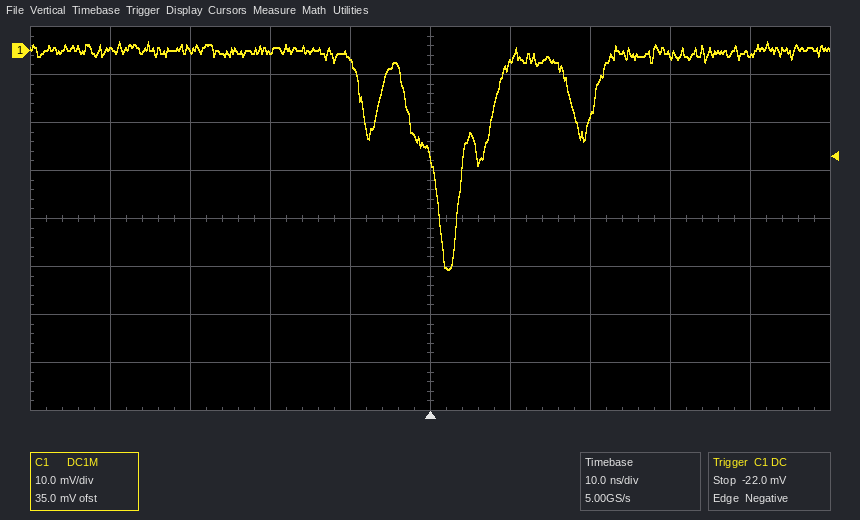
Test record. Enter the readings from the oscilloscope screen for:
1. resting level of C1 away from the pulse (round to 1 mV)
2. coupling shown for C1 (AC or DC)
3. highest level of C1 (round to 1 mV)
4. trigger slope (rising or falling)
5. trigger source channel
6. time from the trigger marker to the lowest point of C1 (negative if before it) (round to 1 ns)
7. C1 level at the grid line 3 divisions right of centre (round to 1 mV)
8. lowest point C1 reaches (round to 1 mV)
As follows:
0 mV
DC
2 mV
falling
C1
+2 ns
-1 mV
-46 mV
